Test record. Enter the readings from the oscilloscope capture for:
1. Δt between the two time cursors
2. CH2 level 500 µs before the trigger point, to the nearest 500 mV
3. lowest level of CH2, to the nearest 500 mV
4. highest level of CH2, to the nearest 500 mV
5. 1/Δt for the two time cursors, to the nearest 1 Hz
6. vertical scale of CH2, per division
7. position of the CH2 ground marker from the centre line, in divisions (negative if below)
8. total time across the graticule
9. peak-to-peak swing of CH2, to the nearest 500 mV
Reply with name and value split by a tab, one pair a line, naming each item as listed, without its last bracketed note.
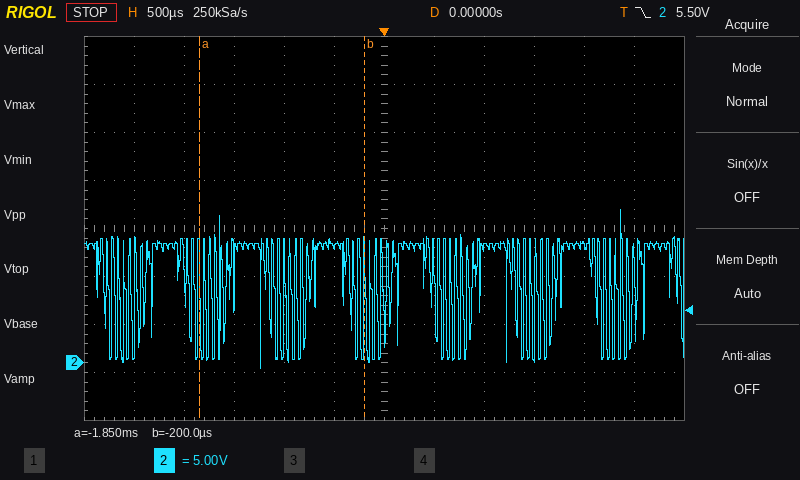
Δt between the two time cursors	1.65 ms
CH2 level 500 µs before the trigger point, to the nearest 500 mV	12.0 V
lowest level of CH2, to the nearest 500 mV	-500 mV
highest level of CH2, to the nearest 500 mV	16.0 V
1/Δt for the two time cursors, to the nearest 1 Hz	606 Hz
vertical scale of CH2, per division	5 V
position of the CH2 ground marker from the centre line, in divisions	-2.8 div
total time across the graticule	6 ms
peak-to-peak swing of CH2, to the nearest 500 mV	16.5 V
